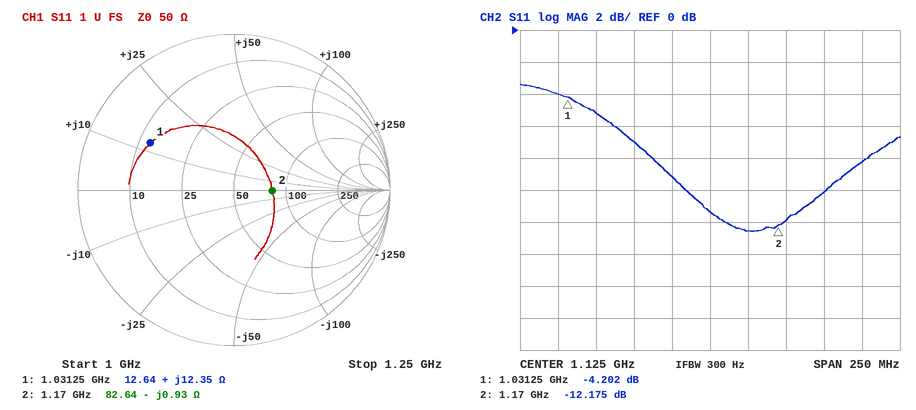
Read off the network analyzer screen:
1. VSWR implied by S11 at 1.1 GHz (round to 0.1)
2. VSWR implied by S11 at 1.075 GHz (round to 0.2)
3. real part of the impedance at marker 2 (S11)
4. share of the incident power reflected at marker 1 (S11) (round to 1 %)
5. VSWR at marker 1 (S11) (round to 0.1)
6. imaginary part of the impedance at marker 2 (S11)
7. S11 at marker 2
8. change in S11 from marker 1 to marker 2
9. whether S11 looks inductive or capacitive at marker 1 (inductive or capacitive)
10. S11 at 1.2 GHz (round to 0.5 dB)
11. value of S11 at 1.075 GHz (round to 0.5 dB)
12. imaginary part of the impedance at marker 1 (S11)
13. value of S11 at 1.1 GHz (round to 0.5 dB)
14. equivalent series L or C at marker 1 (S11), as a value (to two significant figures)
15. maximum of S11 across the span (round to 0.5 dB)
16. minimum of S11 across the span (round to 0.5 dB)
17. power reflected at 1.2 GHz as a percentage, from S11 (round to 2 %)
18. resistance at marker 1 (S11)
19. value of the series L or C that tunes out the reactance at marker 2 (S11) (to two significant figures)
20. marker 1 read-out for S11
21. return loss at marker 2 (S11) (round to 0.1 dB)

2.1
2.6
82.64 Ω
38 %
4.2
-0.93 Ω
-12.175 dB
-7.973 dB
inductive
-10.0 dB
-7.0 dB
+12.35 Ω
-9.0 dB
1.9 nH
-3.5 dB
-12.5 dB
10 %
12.64 Ω
130 pH
-4.202 dB
12.2 dB
